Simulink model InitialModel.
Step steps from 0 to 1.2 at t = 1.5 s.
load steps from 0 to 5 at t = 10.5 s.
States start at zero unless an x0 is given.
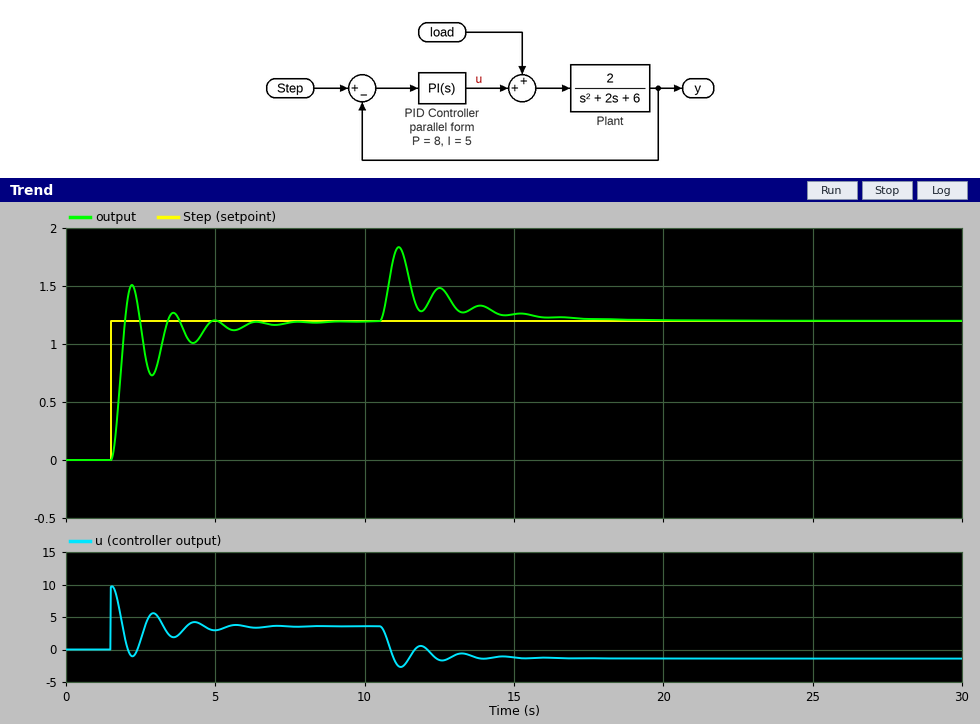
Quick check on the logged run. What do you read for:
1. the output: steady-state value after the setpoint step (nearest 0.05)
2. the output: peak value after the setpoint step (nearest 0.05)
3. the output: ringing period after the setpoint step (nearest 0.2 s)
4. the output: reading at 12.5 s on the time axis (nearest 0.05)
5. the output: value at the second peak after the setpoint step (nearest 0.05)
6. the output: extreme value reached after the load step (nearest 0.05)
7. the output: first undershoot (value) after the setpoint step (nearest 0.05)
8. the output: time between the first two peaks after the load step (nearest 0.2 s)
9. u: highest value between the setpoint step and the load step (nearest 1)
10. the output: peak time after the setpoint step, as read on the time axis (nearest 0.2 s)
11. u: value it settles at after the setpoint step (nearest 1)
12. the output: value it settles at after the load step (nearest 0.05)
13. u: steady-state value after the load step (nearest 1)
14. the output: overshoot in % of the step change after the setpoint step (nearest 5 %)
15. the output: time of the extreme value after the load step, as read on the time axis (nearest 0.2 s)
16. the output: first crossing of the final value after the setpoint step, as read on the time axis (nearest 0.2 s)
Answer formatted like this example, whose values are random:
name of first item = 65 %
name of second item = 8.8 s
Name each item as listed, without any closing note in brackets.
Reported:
the output: steady-state value after the setpoint step = 1.20
the output: peak value after the setpoint step = 1.50
the output: ringing period after the setpoint step = 1.4 s
the output: reading at 12.5 s on the time axis = 1.50
the output: value at the second peak after the setpoint step = 1.25
the output: extreme value reached after the load step = 1.85
the output: first undershoot (value) after the setpoint step = 0.75
the output: time between the first two peaks after the load step = 1.4 s
u: highest value between the setpoint step and the load step = 10
the output: peak time after the setpoint step, as read on the time axis = 2.2 s
u: value it settles at after the setpoint step = 4
the output: value it settles at after the load step = 1.20
u: steady-state value after the load step = -1
the output: overshoot in % of the step change after the setpoint step = 25 %
the output: time of the extreme value after the load step, as read on the time axis = 11.2 s
the output: first crossing of the final value after the setpoint step, as read on the time axis = 2.0 s
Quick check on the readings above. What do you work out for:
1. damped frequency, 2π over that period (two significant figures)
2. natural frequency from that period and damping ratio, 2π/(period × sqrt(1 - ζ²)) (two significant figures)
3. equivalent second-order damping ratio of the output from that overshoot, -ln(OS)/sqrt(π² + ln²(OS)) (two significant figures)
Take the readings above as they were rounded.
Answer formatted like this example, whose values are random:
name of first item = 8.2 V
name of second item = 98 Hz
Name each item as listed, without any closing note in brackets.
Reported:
damped frequency, 2π over that period = 4.5 rad/s
natural frequency from that period and damping ratio, 2π/(period × sqrt(1 - ζ²)) = 4.9 rad/s
equivalent second-order damping ratio of the output from that overshoot, -ln(OS)/sqrt(π² + ln²(OS)) = 0.40
